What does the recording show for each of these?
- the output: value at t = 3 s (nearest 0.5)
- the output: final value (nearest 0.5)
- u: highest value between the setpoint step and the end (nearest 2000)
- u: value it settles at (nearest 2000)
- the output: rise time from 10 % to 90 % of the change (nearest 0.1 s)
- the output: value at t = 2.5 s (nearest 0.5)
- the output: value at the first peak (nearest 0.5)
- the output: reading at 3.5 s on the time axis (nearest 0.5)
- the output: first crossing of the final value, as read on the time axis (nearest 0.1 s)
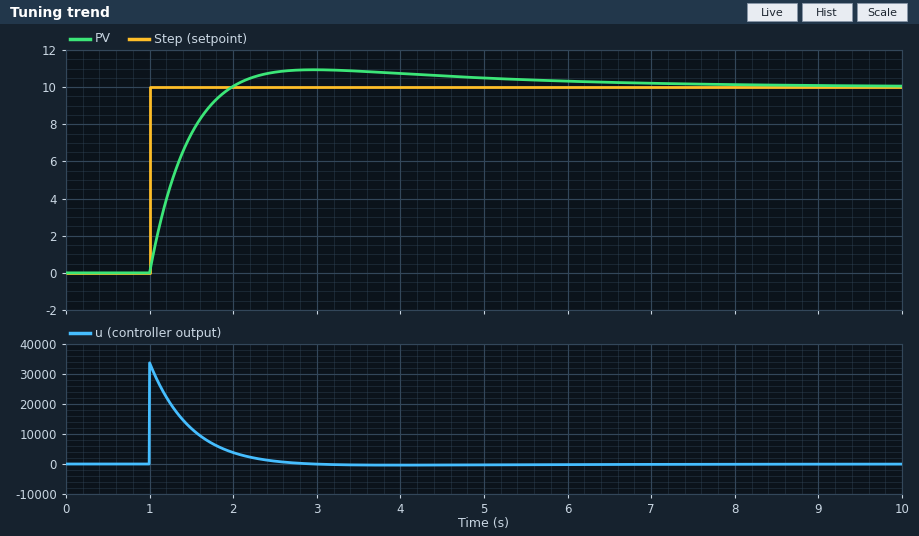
11.0
10.0
34000
0
0.7 s
11.0
11.0
11.0
2.0 s
